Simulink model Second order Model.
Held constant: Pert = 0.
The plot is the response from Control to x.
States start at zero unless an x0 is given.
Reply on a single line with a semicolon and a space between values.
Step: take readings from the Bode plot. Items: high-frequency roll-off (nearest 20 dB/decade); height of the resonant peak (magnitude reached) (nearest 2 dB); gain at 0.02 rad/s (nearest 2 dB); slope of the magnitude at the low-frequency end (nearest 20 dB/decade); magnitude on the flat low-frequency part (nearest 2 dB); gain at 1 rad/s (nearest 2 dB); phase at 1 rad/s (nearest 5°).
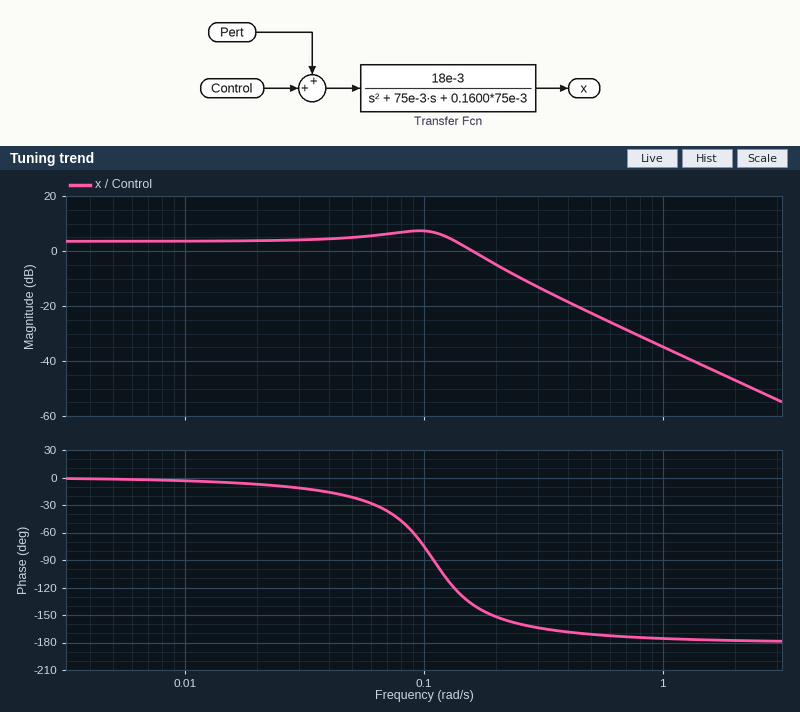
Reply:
-40 dB/decade; 8 dB; 4 dB; 0 dB/decade; 4 dB; -34 dB; -175°
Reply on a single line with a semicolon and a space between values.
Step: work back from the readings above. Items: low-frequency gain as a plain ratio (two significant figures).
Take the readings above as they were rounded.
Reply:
1.6
